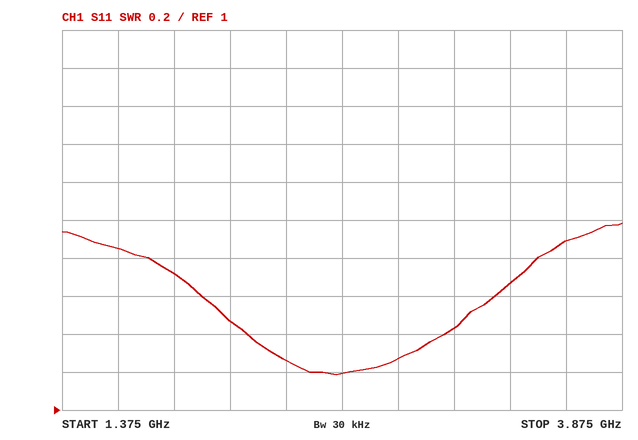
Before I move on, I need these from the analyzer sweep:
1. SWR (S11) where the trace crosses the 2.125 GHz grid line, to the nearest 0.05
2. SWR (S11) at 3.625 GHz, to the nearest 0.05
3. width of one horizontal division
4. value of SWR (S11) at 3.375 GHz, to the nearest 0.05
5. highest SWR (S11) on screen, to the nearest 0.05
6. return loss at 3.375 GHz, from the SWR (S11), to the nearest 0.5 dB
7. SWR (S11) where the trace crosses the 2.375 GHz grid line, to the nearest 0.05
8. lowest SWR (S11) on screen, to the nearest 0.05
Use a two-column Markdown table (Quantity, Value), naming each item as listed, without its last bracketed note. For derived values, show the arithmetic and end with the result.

| Quantity | Value |
|---|---|
| SWR (S11) where the trace crosses the 2.125 GHz grid line, to the nearest 0.05 | 1.45 |
| SWR (S11) at 3.625 GHz, to the nearest 0.05 | 1.90 |
| width of one horizontal division | 250 MHz |
| value of SWR (S11) at 3.375 GHz, to the nearest 0.05 | 1.65 |
| highest SWR (S11) on screen, to the nearest 0.05 | 2.00 |
| return loss at 3.375 GHz, from the SWR (S11), to the nearest 0.5 dB | −20 log10((1.65 − 1)/(1.65 + 1)) ≈ 12.2 dB, so 12.0 dB to the nearest 0.5 dB |
| SWR (S11) where the trace crosses the 2.375 GHz grid line, to the nearest 0.05 | 1.25 |
| lowest SWR (S11) on screen, to the nearest 0.05 | 1.20 |
